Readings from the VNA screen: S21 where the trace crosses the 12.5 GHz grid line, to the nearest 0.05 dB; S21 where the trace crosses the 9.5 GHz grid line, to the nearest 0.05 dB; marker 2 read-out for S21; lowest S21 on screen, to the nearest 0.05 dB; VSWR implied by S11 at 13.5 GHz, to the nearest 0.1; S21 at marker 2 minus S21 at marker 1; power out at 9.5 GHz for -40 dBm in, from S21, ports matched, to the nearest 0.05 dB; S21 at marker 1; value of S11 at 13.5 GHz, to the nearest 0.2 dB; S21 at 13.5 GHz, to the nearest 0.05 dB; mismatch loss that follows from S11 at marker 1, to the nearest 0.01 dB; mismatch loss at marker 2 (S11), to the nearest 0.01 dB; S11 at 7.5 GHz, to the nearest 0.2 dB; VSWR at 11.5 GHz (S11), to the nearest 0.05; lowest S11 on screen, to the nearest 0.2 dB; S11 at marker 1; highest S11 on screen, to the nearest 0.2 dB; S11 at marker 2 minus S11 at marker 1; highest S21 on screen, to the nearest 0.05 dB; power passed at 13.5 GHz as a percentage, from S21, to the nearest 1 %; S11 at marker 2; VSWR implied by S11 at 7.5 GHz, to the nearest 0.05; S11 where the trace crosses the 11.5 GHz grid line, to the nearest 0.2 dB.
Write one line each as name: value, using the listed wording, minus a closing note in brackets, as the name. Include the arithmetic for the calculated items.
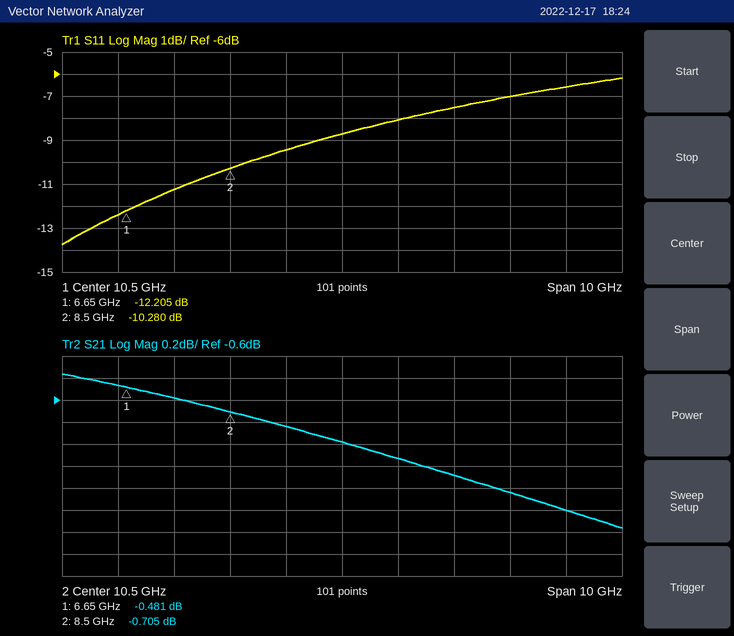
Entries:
S21 where the trace crosses the 12.5 GHz grid line, to the nearest 0.05 dB: -1.30 dB
S21 where the trace crosses the 9.5 GHz grid line, to the nearest 0.05 dB: -0.85 dB
marker 2 read-out for S21: -0.705 dB
lowest S21 on screen, to the nearest 0.05 dB: -1.75 dB
VSWR implied by S11 at 13.5 GHz, to the nearest 0.1: |Γ| = 10^(-7/20) = 0.4467; VSWR = (1 + 0.4467)/(1 − 0.4467) ≈ 2.6
S21 at marker 2 minus S21 at marker 1: -0.705 − (-0.481) = -0.224 dB
power out at 9.5 GHz for -40 dBm in, from S21, ports matched, to the nearest 0.05 dB: -40 dBm + (-0.85 dB) = -40.85 dBm
S21 at marker 1: -0.481 dB
value of S11 at 13.5 GHz, to the nearest 0.2 dB: -7.0 dB
S21 at 13.5 GHz, to the nearest 0.05 dB: -1.45 dB
mismatch loss that follows from S11 at marker 1, to the nearest 0.01 dB: −10 log10(1 − 10^(-12.205/10)) ≈ 0.27 dB
mismatch loss at marker 2 (S11), to the nearest 0.01 dB: −10 log10(1 − 10^(-10.28/10)) ≈ 0.43 dB
S11 at 7.5 GHz, to the nearest 0.2 dB: -11.2 dB
VSWR at 11.5 GHz (S11), to the nearest 0.05: |Γ| = 10^(-8/20) = 0.3981; VSWR = (1 + 0.3981)/(1 − 0.3981) ≈ 2.32, so 2.30 to the nearest 0.05
lowest S11 on screen, to the nearest 0.2 dB: -13.8 dB
S11 at marker 1: -12.205 dB
highest S11 on screen, to the nearest 0.2 dB: -6.2 dB
S11 at marker 2 minus S11 at marker 1: -10.28 − (-12.205) = 1.925 dB
highest S21 on screen, to the nearest 0.05 dB: -0.35 dB
power passed at 13.5 GHz as a percentage, from S21, to the nearest 1 %: 10^(-1.45/10) ≈ 72 %
S11 at marker 2: -10.280 dB
VSWR implied by S11 at 7.5 GHz, to the nearest 0.05: |Γ| = 10^(-11.2/20) = 0.2754; VSWR = (1 + 0.2754)/(1 − 0.2754) ≈ 1.76, so 1.75 to the nearest 0.05
S11 where the trace crosses the 11.5 GHz grid line, to the nearest 0.2 dB: -8.0 dB
